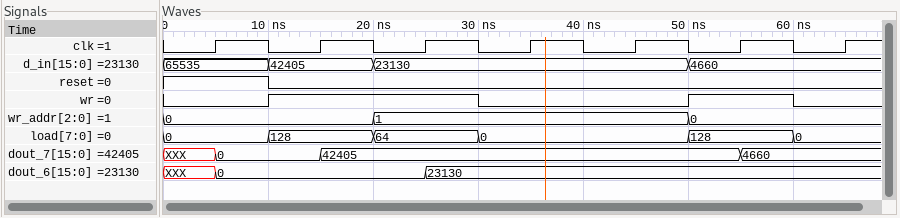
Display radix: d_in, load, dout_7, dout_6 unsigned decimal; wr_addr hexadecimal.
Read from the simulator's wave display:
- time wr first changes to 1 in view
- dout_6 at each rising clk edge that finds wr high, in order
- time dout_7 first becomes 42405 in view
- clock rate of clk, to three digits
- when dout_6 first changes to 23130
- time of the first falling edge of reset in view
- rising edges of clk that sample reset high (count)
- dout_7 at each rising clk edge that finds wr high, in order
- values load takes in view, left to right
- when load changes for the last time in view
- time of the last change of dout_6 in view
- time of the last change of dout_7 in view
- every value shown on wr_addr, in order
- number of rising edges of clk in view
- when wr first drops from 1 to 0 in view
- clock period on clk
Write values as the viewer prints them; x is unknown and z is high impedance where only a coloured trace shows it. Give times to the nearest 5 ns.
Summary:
10 ns
0, 0, 23130
15 ns
100 MHz
25 ns
10 ns
1
0, 42405, 42405
0, 128, 64, 0, 128, 0
60 ns
25 ns
55 ns
0, 1, 0
7
30 ns
10 ns
